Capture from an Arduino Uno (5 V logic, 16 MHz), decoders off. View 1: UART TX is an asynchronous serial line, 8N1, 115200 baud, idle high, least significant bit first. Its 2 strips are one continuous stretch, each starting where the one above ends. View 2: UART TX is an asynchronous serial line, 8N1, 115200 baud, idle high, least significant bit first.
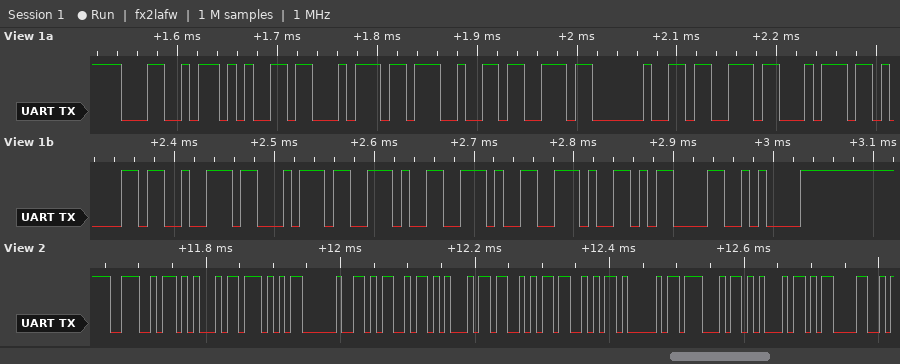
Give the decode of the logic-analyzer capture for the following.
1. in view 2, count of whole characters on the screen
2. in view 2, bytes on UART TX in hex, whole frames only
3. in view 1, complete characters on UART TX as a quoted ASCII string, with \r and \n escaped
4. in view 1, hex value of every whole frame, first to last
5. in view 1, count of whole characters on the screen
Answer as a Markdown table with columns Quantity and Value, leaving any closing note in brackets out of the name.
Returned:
| Quantity | Value |
|---|---|
| in view 2, count of whole characters on the screen | 12 |
| in view 2, bytes on UART TX in hex, whole frames only | 0x4E 0x45 0x57 0x20 0x4D 0x45 0x53 0x53 0x41 0x47 0x45 0x0D |
| in view 1, complete characters on UART TX as a quoted ASCII string, with \r and \n escaped | "Let's start...\r\n" |
| in view 1, hex value of every whole frame, first to last | 4C 65 74 27 73 20 73 74 61 72 74 2E 2E 2E 0D 0A |
| in view 1, count of whole characters on the screen | 16 |
